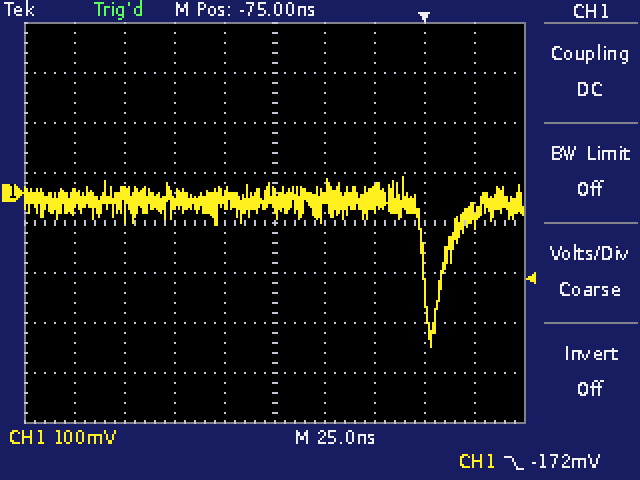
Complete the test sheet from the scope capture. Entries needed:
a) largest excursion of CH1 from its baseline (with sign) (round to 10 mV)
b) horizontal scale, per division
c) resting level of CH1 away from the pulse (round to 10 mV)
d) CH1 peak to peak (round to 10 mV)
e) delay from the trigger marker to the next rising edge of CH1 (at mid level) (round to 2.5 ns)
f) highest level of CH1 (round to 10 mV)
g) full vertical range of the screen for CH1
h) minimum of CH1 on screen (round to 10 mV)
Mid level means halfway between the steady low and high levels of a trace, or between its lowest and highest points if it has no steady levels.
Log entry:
-290 mV
25 ns
-20 mV
340 mV
10.0 ns
30 mV
800 mV
-310 mV
